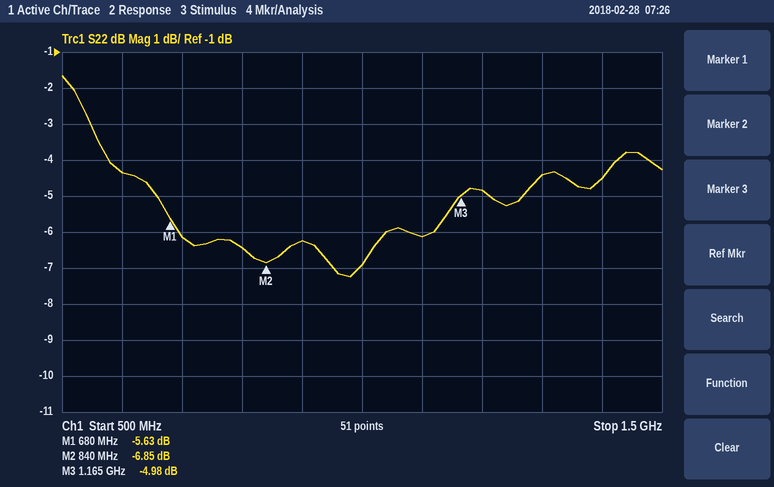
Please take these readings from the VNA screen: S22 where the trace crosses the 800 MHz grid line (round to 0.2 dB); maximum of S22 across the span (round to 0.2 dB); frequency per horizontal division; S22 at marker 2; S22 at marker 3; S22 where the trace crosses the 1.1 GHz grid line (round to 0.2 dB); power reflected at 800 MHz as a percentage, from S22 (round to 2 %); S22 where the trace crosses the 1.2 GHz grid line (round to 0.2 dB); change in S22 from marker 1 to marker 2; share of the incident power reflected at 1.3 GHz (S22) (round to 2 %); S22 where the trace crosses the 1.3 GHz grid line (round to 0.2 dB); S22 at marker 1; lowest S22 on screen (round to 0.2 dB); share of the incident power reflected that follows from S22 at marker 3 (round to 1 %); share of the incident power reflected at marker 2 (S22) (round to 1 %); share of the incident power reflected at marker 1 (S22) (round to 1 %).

-6.4 dB
-1.6 dB
100 MHz
-6.85 dB
-4.98 dB
-6.2 dB
22 %
-4.8 dB
-1.22 dB
36 %
-4.4 dB
-5.63 dB
-7.2 dB
32 %
21 %
27 %
